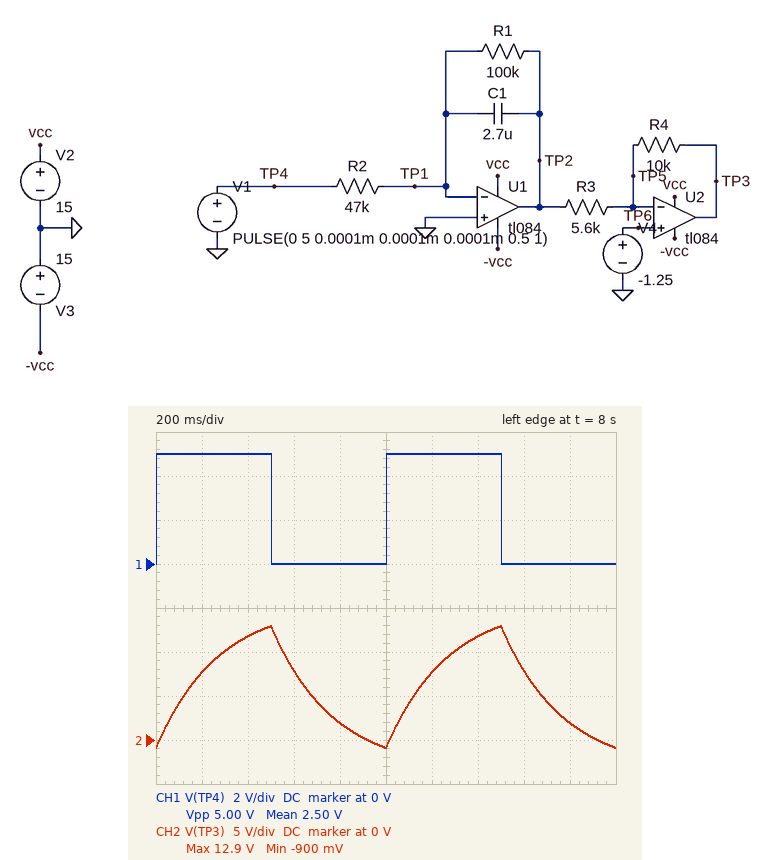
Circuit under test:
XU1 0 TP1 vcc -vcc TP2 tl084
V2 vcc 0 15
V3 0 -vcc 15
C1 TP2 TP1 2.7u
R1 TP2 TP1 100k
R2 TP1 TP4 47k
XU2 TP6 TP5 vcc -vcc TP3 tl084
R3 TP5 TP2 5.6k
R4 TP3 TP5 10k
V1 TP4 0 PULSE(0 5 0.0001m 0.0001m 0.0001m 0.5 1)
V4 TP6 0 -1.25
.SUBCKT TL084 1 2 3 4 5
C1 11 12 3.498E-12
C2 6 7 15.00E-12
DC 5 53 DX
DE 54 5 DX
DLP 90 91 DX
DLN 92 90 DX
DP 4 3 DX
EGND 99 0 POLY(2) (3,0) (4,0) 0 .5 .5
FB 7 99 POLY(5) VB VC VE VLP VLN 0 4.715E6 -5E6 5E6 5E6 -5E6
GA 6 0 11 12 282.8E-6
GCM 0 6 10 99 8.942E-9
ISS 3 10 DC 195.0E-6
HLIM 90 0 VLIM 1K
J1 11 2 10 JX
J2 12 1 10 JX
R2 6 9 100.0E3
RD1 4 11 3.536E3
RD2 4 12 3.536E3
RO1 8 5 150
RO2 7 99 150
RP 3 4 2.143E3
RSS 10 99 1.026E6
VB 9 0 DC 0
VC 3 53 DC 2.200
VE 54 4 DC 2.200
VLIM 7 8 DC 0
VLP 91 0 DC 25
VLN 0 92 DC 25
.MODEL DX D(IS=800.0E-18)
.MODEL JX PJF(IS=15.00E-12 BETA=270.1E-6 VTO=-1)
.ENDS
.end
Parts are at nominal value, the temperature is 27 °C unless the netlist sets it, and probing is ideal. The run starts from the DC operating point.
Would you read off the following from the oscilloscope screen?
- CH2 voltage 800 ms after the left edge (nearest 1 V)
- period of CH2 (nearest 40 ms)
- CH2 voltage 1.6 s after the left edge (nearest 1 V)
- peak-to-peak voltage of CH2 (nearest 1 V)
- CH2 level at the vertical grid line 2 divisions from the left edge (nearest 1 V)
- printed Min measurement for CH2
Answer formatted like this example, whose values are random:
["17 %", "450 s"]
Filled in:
["2 V", "1.00 s", "8 V", "14 V", "12 V", "-900 mV"]
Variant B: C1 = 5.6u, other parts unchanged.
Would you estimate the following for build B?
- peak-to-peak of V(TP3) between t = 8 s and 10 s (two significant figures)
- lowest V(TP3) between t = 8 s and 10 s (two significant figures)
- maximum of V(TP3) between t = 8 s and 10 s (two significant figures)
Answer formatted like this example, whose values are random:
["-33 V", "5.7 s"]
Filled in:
["8.0 V", "2.0 V", "10 V"]
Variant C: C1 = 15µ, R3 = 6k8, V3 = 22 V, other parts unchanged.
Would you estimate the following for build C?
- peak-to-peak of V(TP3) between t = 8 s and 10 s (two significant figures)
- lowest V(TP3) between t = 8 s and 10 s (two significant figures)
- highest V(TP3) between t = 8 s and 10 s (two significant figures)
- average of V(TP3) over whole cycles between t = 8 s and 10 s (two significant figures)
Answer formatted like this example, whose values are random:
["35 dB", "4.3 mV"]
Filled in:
["2.6 V", "3.4 V", "6.0 V", "4.7 V"]
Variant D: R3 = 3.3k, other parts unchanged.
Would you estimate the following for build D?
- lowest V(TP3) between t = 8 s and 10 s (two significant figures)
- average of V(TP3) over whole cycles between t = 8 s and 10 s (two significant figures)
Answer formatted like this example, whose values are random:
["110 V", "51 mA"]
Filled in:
["-670 mV", "8.9 V"]
